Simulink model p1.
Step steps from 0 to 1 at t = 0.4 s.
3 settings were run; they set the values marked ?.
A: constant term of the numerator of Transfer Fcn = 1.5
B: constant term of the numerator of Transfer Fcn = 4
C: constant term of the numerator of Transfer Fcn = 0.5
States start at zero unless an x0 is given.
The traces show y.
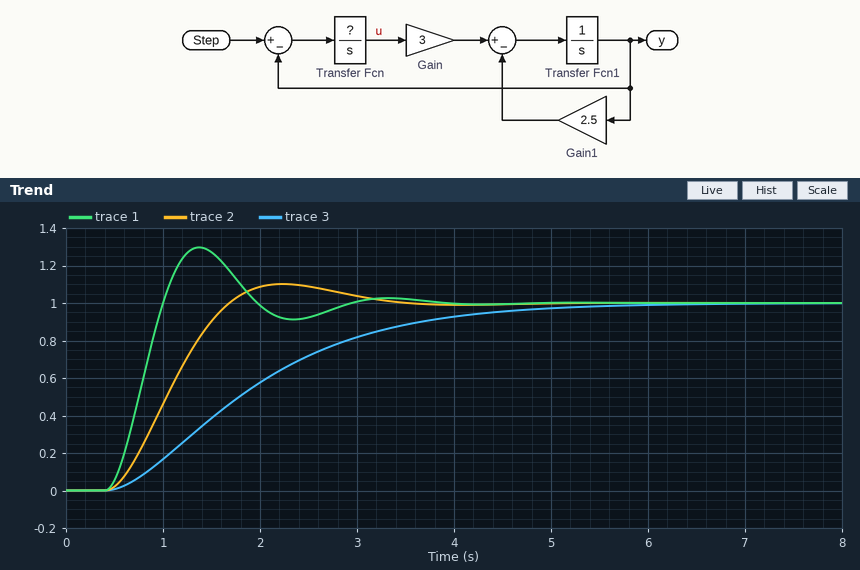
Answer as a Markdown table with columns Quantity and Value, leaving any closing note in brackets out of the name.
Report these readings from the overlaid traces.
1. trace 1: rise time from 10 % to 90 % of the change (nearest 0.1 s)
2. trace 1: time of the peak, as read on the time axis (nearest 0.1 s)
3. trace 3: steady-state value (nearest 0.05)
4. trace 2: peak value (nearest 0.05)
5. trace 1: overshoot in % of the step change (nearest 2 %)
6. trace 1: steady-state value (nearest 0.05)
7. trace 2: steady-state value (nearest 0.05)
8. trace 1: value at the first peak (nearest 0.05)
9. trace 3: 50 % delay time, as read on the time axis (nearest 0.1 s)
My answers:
| Quantity | Value |
|---|---|
| trace 1: rise time from 10 % to 90 % of the change | 0.4 s |
| trace 1: time of the peak, as read on the time axis | 1.4 s |
| trace 3: steady-state value | 1.00 |
| trace 2: peak value | 1.10 |
| trace 1: overshoot in % of the step change | 30 % |
| trace 1: steady-state value | 1.00 |
| trace 2: steady-state value | 1.00 |
| trace 1: value at the first peak | 1.30 |
| trace 3: 50 % delay time, as read on the time axis | 1.8 s |
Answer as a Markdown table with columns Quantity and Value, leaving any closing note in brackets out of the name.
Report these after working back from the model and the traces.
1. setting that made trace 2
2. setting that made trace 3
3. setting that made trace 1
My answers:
| Quantity | Value |
|---|---|
| setting that made trace 2 | A |
| setting that made trace 3 | C |
| setting that made trace 1 | B |
